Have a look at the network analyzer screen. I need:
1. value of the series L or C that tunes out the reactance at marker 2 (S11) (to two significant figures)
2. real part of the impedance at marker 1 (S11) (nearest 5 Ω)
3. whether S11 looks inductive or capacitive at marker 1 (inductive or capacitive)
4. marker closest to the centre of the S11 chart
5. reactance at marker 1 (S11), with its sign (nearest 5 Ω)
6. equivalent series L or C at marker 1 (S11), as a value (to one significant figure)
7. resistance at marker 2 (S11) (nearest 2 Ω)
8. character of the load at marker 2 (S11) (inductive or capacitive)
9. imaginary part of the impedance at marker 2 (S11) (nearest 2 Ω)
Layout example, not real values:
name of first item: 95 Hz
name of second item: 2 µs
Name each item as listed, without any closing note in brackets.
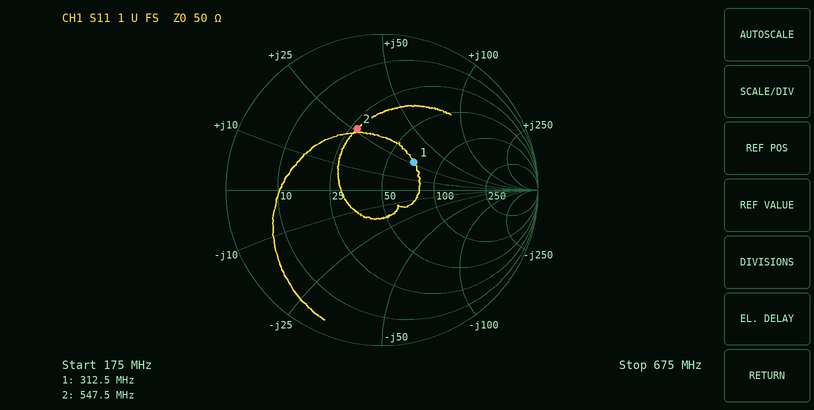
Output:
value of the series L or C that tunes out the reactance at marker 2 (S11): 11 pF
real part of the impedance at marker 1 (S11): 70 Ω
whether S11 looks inductive or capacitive at marker 1: inductive
marker closest to the centre of the S11 chart: marker 1
reactance at marker 1 (S11), with its sign: +25 Ω
equivalent series L or C at marker 1 (S11), as a value: 10 nH
resistance at marker 2 (S11): 28 Ω
character of the load at marker 2 (S11): inductive
imaginary part of the impedance at marker 2 (S11): +26 Ω
